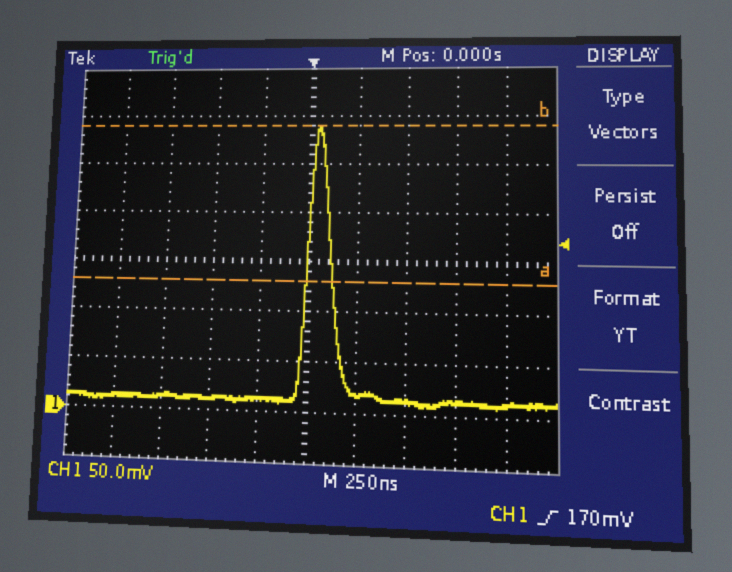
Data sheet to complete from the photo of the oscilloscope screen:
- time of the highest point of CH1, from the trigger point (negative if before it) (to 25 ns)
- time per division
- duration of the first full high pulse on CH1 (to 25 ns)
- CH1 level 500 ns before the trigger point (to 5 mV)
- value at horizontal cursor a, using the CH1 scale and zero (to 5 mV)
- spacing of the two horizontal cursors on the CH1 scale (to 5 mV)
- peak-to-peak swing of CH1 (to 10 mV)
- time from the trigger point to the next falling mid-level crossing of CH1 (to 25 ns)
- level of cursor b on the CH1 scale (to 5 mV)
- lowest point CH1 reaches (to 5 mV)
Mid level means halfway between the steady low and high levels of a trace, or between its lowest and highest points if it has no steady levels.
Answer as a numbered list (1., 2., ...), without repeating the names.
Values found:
1. +50 ns
2. 250 ns
3. 125 ns
4. 10 mV
5. 130 mV
6. 160 mV
7. 280 mV
8. 125 ns
9. 290 mV
10. 10 mV
